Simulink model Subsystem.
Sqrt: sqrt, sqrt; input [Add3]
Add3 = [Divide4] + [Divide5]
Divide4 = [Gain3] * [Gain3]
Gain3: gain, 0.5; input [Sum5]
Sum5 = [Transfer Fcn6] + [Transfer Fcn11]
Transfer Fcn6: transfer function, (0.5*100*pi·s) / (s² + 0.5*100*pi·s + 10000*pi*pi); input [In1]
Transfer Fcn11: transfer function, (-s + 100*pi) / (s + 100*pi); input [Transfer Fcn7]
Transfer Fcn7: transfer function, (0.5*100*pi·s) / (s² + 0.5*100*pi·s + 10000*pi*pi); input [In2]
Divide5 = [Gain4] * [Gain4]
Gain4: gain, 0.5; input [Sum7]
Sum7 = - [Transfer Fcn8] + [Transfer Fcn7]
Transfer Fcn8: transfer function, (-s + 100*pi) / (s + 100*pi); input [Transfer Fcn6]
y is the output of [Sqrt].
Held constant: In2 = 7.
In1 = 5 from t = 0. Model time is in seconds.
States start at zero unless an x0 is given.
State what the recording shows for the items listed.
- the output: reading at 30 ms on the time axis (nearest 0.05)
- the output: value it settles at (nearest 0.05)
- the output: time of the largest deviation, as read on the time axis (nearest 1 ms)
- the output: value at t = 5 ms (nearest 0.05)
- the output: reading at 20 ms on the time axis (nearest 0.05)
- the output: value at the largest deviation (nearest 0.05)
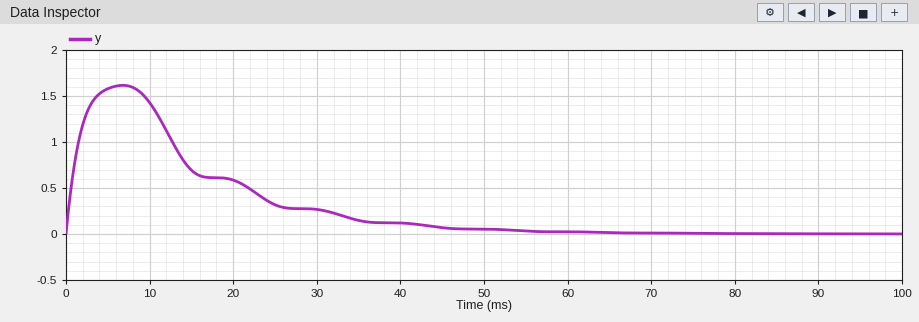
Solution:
0.25
0.00
7 ms
1.60
0.60
1.60
